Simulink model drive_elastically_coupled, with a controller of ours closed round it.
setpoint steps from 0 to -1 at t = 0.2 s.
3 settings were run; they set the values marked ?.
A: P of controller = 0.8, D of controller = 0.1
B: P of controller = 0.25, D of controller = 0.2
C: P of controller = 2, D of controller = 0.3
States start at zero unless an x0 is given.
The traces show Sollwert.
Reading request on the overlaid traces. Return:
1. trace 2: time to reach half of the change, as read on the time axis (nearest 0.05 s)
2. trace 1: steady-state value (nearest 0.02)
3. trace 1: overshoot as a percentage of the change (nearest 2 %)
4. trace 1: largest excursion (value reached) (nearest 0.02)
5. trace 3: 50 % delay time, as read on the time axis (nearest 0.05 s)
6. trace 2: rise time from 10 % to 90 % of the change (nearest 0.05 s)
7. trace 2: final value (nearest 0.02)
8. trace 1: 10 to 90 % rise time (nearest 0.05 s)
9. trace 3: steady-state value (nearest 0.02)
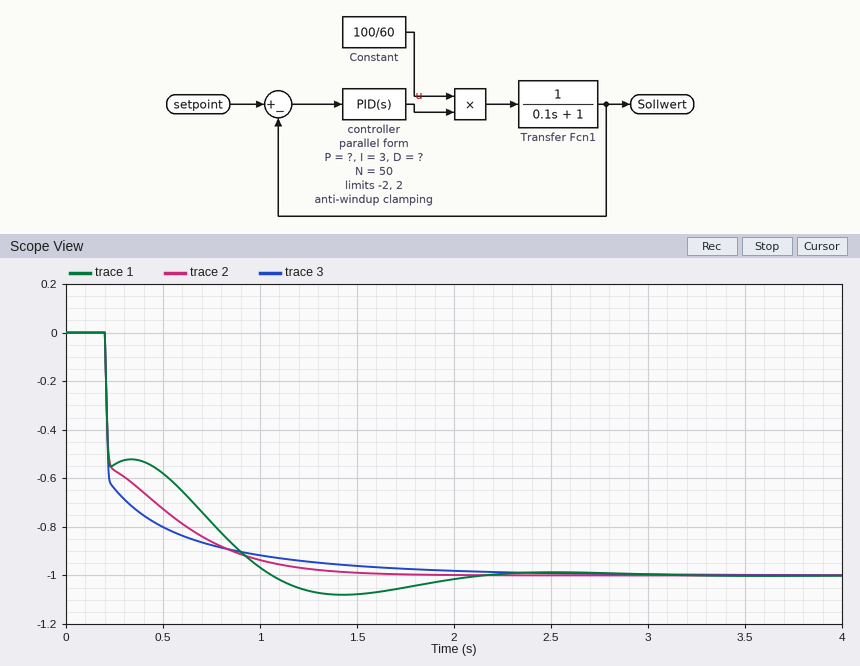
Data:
0.20 s
-1.00
8 %
-1.08
0.20 s
0.65 s
-1.00
0.70 s
-1.00
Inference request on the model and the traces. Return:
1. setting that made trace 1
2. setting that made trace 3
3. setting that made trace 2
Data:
B
C
A
